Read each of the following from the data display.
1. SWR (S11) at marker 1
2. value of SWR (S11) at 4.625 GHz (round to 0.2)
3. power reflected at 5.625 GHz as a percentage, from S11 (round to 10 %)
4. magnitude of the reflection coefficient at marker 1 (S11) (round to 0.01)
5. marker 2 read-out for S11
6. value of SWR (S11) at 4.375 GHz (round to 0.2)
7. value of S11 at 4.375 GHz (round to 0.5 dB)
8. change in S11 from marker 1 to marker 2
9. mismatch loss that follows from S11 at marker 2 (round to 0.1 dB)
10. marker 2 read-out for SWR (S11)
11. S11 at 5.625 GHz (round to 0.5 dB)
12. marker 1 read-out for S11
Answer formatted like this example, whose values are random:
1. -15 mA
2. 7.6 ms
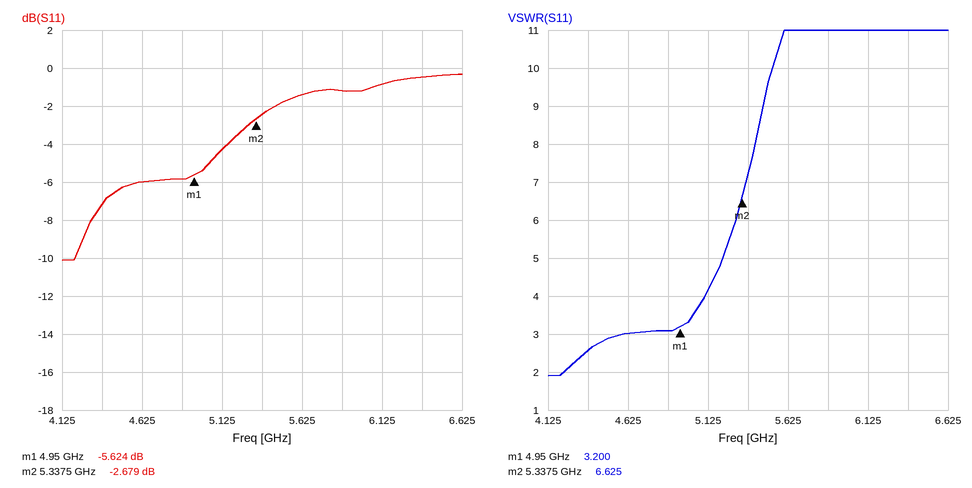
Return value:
1. 3.200
2. 3.0
3. 70 %
4. 0.52
5. -2.679 dB
6. 2.6
7. -7.0 dB
8. 2.945 dB
9. 3.4 dB
10. 6.625
11. -1.5 dB
12. -5.624 dB
